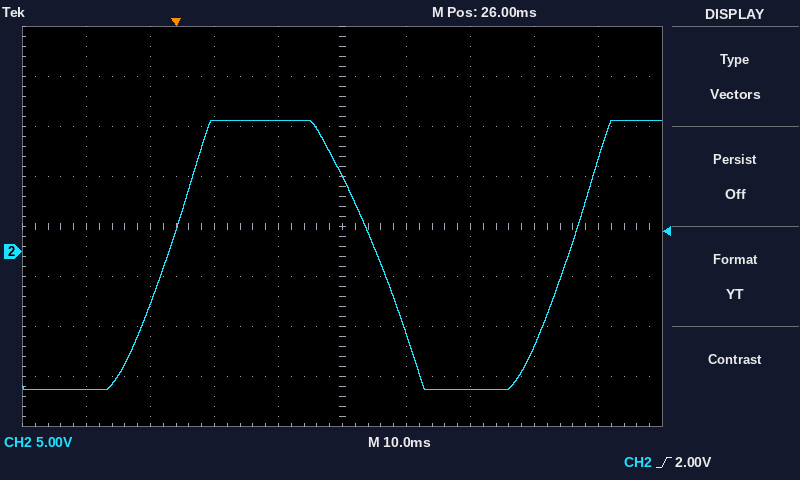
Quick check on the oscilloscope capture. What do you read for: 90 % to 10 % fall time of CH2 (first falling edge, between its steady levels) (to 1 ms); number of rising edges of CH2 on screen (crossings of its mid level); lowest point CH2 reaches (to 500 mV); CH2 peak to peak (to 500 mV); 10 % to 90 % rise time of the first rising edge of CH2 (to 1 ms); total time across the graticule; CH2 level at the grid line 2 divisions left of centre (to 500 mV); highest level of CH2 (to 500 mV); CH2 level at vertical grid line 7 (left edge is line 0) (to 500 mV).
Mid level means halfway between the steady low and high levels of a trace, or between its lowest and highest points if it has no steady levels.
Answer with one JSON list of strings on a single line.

["14 ms", "2", "-14.0 V", "27.0 V", "12 ms", "100 ms", "13.0 V", "13.0 V", "-14.0 V"]
